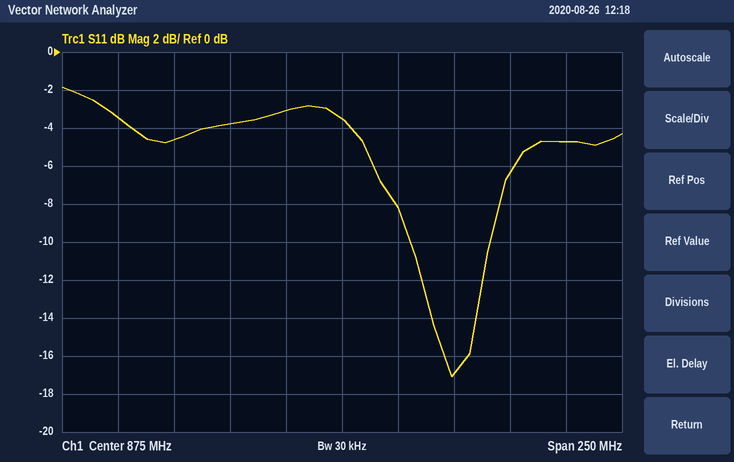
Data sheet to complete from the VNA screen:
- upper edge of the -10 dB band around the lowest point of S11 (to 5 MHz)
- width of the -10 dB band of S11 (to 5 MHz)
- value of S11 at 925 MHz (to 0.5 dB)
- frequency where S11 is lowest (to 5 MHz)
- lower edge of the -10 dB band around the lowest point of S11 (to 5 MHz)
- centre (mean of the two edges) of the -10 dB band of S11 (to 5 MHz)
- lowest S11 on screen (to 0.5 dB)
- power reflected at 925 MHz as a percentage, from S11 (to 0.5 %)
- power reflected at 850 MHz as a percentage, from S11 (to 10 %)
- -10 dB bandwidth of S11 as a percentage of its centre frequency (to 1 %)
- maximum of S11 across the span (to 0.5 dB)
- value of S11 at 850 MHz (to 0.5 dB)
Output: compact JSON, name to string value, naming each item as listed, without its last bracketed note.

{"upper edge of the -10 dB band around the lowest point of S11": "940 MHz", "width of the -10 dB band of S11": "35 MHz", "value of S11 at 925 MHz": "-17.0 dB", "frequency where S11 is lowest": "925 MHz", "lower edge of the -10 dB band around the lowest point of S11": "905 MHz", "centre (mean of the two edges) of the -10 dB band of S11": "925 MHz", "lowest S11 on screen": "-17.0 dB", "power reflected at 925 MHz as a percentage, from S11": "2.0 %", "power reflected at 850 MHz as a percentage, from S11": "50 %", "-10 dB bandwidth of S11 as a percentage of its centre frequency": "4 %", "maximum of S11 across the span": "-2.0 dB", "value of S11 at 850 MHz": "-3.0 dB"}
